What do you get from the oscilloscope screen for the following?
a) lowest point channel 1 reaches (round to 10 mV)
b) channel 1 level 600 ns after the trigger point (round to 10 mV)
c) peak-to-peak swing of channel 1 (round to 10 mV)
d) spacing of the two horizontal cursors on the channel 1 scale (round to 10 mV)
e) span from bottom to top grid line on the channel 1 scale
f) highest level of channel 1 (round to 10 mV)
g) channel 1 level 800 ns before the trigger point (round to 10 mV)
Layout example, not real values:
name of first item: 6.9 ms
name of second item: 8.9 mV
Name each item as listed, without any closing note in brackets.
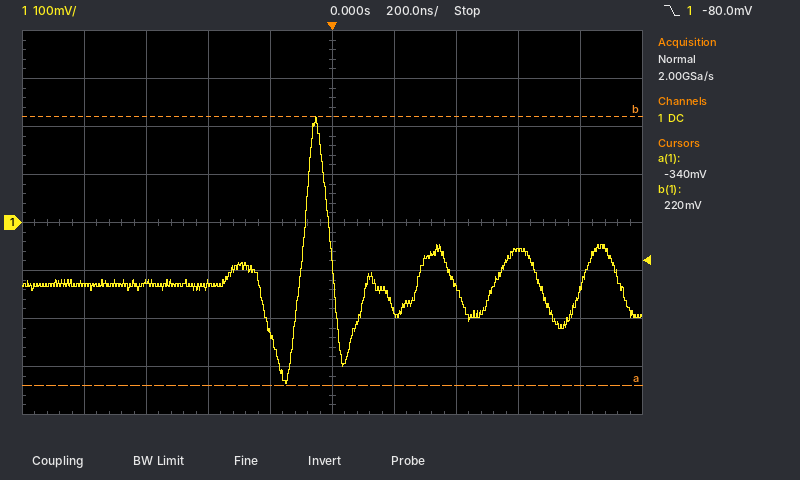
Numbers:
lowest point channel 1 reaches: -340 mV
channel 1 level 600 ns after the trigger point: -60 mV
peak-to-peak swing of channel 1: 560 mV
spacing of the two horizontal cursors on the channel 1 scale: 560 mV
span from bottom to top grid line on the channel 1 scale: 800 mV
highest level of channel 1: 220 mV
channel 1 level 800 ns before the trigger point: -130 mV
